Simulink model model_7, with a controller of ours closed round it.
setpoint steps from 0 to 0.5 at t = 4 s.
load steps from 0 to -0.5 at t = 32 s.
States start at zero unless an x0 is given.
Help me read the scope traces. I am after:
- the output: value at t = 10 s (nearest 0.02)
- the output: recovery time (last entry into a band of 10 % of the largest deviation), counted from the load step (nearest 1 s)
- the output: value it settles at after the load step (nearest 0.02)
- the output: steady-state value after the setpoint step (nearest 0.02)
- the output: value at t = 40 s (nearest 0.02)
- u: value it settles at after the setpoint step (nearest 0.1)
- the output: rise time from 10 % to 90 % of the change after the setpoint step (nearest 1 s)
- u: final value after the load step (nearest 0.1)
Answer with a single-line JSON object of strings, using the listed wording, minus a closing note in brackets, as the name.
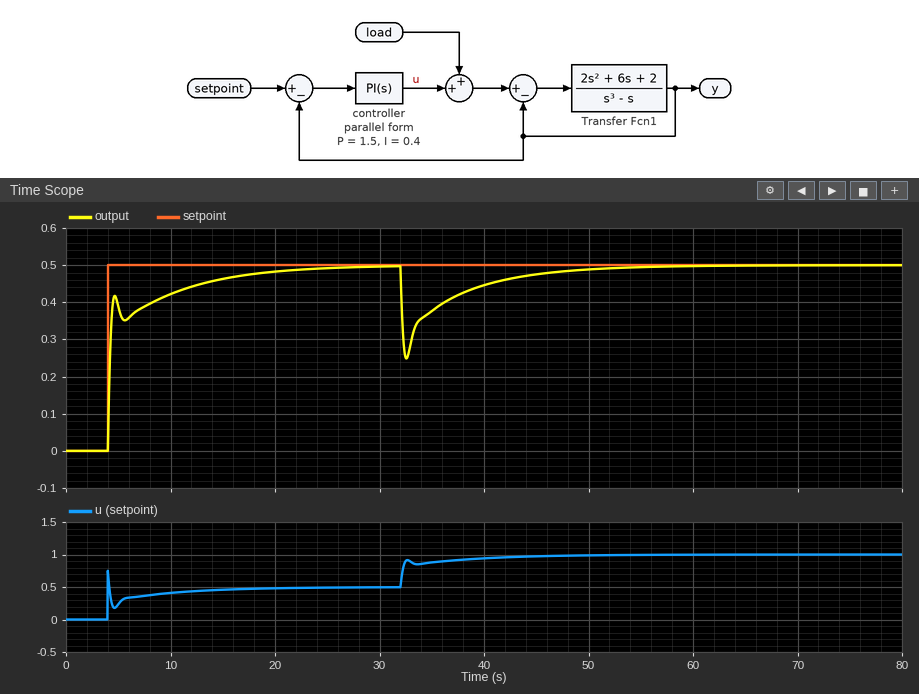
{"the output: value at t = 10 s": "0.42", "the output: recovery time (last entry into a band of 10 % of the largest deviation), counted from the load step": "13 s", "the output: value it settles at after the load step": "0.50", "the output: steady-state value after the setpoint step": "0.50", "the output: value at t = 40 s": "0.44", "u: value it settles at after the setpoint step": "0.5", "the output: rise time from 10 % to 90 % of the change after the setpoint step": "9 s", "u: final value after the load step": "1.0"}
